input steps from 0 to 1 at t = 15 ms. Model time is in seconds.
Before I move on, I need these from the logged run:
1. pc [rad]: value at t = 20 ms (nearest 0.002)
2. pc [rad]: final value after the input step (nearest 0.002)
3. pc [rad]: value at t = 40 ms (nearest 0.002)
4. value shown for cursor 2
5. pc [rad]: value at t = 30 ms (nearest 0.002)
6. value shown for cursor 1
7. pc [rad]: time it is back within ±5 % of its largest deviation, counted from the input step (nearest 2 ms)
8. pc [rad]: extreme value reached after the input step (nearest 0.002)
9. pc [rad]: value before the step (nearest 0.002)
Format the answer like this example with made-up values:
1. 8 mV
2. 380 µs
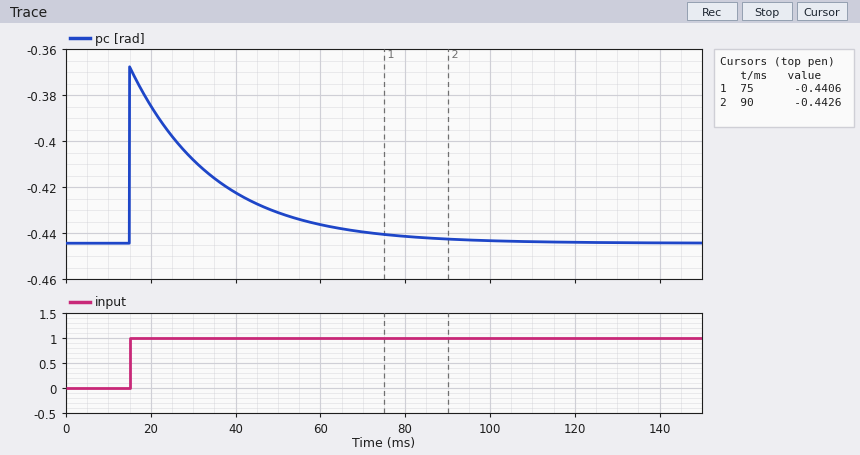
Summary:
1. -0.384
2. -0.444
3. -0.422
4. -0.4426
5. -0.408
6. -0.4406
7. 60 ms
8. -0.368
9. -0.444
